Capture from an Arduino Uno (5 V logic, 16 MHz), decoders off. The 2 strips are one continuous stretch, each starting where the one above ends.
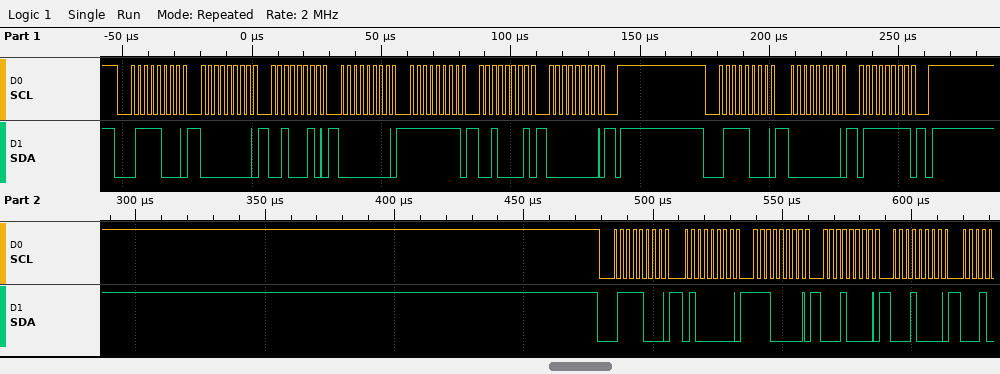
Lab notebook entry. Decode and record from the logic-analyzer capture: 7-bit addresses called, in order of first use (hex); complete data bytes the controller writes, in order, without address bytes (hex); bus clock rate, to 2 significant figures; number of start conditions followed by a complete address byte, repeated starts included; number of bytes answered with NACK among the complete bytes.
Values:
0x3C
00 22 00 FF 21 00 00 7F 40 E0 10 10
400 kHz
3
0
